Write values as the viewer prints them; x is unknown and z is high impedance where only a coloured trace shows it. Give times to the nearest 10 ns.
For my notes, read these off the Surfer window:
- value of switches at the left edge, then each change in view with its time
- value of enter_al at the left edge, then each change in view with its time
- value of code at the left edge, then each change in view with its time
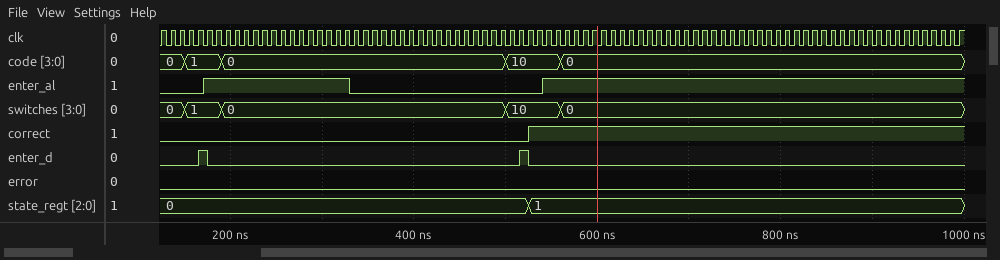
0, 1 at 150 ns, 0 at 190 ns, 10 at 500 ns, 0 at 560 ns
0, 1 at 170 ns, 0 at 330 ns, 1 at 540 ns
0, 1 at 150 ns, 0 at 190 ns, 10 at 500 ns, 0 at 560 ns
